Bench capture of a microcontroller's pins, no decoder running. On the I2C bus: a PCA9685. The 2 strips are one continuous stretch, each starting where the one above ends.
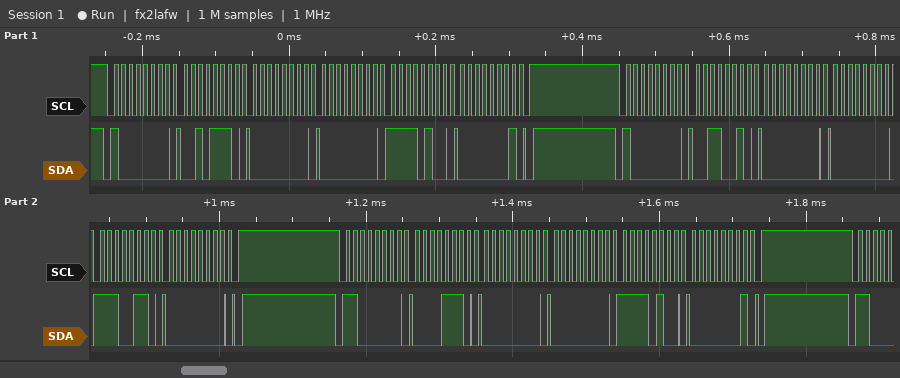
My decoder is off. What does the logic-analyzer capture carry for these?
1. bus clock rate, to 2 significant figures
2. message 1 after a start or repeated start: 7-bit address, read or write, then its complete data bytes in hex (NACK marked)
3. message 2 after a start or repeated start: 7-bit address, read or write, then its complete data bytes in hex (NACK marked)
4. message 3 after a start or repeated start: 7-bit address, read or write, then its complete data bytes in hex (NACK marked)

100 kHz
0x40 write: 2E 00 00 F4 01
0x40 write: 32 00 00 E6 00
0x60 write: 0E 00 00 F4 01
